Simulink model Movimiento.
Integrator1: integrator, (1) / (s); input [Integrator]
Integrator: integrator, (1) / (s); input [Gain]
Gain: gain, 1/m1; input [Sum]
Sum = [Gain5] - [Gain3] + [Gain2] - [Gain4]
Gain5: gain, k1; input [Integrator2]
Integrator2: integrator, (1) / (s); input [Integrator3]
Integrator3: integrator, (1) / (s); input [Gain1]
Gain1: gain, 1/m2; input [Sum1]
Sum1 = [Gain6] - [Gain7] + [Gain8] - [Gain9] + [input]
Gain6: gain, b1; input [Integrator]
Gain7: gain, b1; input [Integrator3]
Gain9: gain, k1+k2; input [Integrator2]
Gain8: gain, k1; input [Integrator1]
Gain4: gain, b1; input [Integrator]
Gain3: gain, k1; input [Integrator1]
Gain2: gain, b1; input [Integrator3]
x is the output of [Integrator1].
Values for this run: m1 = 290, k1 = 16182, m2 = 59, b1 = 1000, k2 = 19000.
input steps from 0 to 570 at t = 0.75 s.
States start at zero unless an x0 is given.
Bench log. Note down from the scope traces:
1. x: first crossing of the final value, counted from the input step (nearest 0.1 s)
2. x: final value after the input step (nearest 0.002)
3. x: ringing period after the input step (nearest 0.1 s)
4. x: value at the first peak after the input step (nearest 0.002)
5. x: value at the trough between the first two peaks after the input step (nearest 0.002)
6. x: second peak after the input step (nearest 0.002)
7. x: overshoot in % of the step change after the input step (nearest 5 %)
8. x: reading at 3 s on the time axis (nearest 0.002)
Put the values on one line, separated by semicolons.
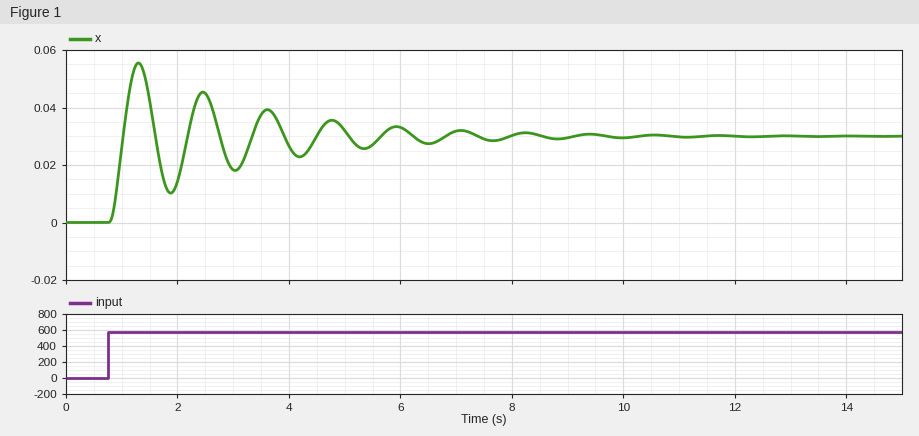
0.3 s; 0.030; 1.2 s; 0.056; 0.010; 0.046; 85 %; 0.018
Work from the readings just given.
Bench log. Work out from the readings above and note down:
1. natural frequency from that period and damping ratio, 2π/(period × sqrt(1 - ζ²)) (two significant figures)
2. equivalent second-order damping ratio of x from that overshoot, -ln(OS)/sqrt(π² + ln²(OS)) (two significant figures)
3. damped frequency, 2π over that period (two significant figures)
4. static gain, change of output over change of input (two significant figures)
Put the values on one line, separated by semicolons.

5.2 rad/s; 0.052; 5.2 rad/s; 0.000053
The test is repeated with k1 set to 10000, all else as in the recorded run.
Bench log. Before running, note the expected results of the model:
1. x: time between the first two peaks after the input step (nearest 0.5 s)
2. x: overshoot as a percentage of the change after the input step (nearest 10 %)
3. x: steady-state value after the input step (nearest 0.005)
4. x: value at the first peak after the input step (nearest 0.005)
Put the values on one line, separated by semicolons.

1.5 s; 70 %; 0.030; 0.050
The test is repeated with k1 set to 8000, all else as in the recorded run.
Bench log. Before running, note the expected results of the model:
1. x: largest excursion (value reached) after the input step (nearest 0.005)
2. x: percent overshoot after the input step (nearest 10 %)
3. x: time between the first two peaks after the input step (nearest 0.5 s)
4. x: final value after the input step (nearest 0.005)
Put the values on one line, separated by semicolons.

0.050; 70 %; 1.5 s; 0.030
